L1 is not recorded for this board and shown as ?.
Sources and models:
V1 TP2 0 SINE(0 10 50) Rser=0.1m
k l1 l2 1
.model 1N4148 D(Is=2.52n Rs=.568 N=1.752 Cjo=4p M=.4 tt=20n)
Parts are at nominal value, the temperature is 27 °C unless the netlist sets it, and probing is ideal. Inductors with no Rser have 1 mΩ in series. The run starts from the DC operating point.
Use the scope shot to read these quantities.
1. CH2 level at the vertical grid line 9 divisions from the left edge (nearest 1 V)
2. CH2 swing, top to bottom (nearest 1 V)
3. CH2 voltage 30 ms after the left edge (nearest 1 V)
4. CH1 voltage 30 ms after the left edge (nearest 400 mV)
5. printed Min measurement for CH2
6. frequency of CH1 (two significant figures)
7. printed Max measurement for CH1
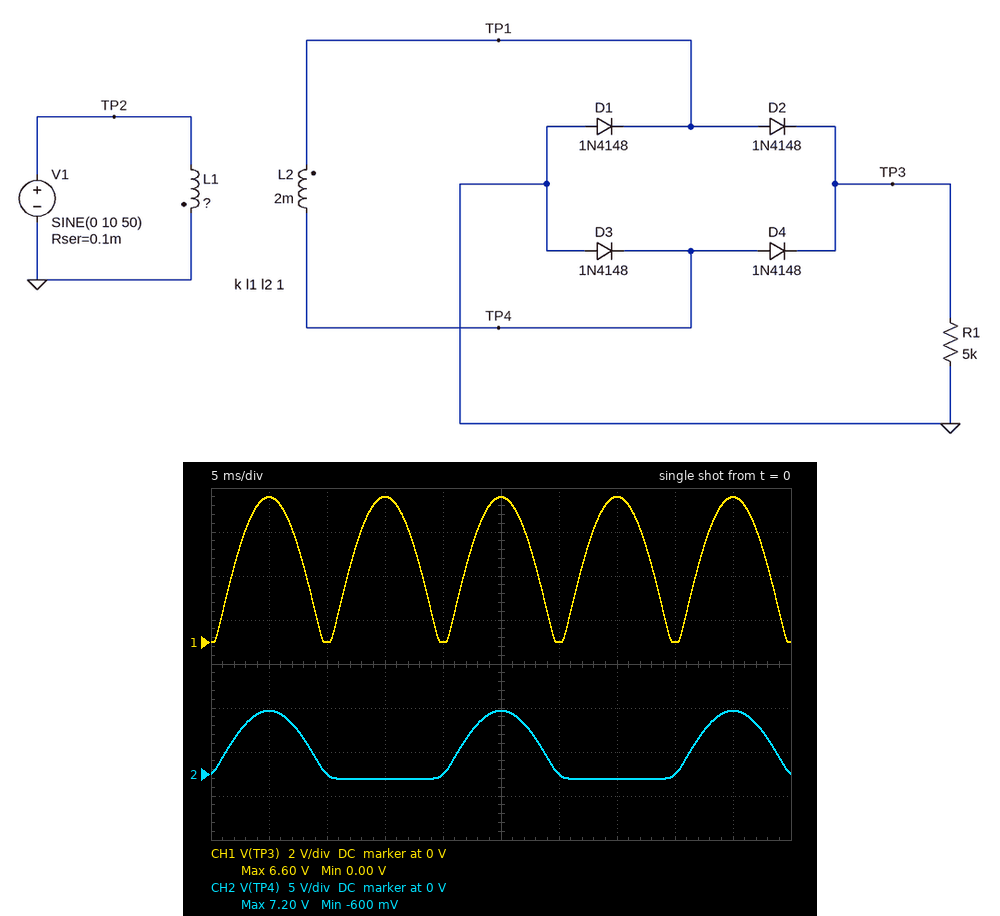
7 V
8 V
0 V
0 V
-600 mV
100 Hz
6.60 V
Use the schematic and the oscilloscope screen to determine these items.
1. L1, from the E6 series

3.3 mH
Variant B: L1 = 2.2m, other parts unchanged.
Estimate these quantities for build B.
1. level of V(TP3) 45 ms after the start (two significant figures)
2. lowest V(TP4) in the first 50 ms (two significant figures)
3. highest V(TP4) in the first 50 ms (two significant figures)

8.3 V
-610 mV
8.9 V
